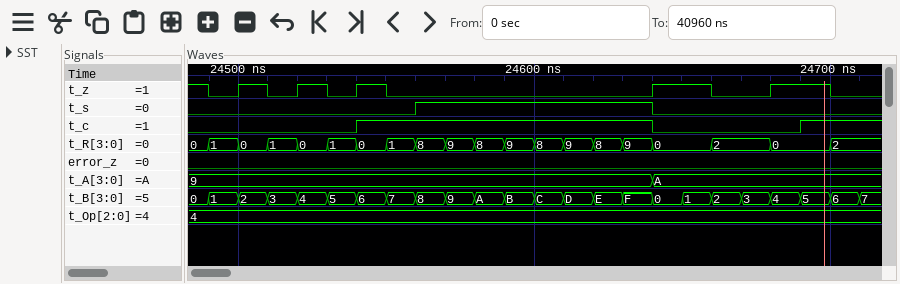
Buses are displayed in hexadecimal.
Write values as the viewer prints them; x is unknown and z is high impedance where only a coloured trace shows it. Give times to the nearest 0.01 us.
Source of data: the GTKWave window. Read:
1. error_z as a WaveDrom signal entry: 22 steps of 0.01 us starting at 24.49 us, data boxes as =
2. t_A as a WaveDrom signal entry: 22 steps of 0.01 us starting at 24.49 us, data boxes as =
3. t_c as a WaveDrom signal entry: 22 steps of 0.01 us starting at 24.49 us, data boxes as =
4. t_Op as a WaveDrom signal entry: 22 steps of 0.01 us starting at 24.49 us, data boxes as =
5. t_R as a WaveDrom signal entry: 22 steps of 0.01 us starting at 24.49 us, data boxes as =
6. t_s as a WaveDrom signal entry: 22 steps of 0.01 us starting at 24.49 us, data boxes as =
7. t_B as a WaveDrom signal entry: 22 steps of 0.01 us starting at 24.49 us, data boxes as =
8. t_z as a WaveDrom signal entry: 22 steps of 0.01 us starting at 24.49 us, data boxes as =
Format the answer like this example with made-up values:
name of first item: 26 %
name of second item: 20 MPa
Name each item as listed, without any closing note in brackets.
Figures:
error_z as a WaveDrom signal entry: 22 steps of 0.01 us starting at 24.49 us, data boxes as =: {name: 'error_z', wave: '0.....................'}
t_A as a WaveDrom signal entry: 22 steps of 0.01 us starting at 24.49 us, data boxes as =: {name: 't_A', wave: '=..............=......', data: '9 A'}
t_c as a WaveDrom signal entry: 22 steps of 0.01 us starting at 24.49 us, data boxes as =: {name: 't_c', wave: '0....1.........0....1.'}
t_Op as a WaveDrom signal entry: 22 steps of 0.01 us starting at 24.49 us, data boxes as =: {name: 't_Op', wave: '=.....................', data: '4'}
t_R as a WaveDrom signal entry: 22 steps of 0.01 us starting at 24.49 us, data boxes as =: {name: 't_R', wave: '================.=.=.=', data: '1 0 1 0 1 0 1 8 9 8 9 8 9 8 9 0 2 0 2'}
t_s as a WaveDrom signal entry: 22 steps of 0.01 us starting at 24.49 us, data boxes as =: {name: 't_s', wave: '0......1.......0......'}
t_B as a WaveDrom signal entry: 22 steps of 0.01 us starting at 24.49 us, data boxes as =: {name: 't_B', wave: '======================', data: '1 2 3 4 5 6 7 8 9 A B C D E F 0 1 2 3 4 5 6'}
t_z as a WaveDrom signal entry: 22 steps of 0.01 us starting at 24.49 us, data boxes as =: {name: 't_z', wave: '0101010........1.0.1.0'}
